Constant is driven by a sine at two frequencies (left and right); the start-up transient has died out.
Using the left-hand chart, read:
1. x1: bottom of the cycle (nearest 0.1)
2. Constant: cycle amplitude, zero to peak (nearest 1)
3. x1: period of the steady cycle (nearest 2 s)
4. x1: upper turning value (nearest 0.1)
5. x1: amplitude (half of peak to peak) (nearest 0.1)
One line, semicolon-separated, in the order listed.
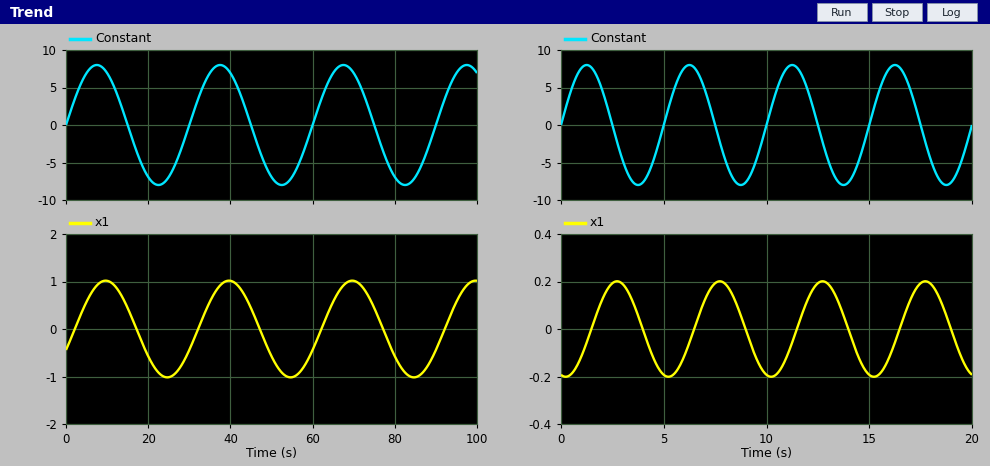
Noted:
-1.0; 8; 30 s; 1.0; 1.0
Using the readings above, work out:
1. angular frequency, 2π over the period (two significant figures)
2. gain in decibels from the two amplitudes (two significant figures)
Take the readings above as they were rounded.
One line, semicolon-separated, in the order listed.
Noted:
0.21 rad/s; -18 dB
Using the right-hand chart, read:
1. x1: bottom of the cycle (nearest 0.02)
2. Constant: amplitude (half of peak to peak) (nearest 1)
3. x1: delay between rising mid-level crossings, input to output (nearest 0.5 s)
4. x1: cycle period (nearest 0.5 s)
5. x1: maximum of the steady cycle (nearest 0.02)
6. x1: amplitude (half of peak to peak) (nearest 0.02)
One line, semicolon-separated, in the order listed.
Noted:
-0.20; 8; 1.5 s; 5.0 s; 0.20; 0.20
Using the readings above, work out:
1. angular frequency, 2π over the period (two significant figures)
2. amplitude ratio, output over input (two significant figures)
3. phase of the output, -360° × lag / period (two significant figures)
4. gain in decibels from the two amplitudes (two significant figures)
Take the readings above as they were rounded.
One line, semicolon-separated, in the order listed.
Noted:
1.3 rad/s; 0.025; -110°; -32 dB
